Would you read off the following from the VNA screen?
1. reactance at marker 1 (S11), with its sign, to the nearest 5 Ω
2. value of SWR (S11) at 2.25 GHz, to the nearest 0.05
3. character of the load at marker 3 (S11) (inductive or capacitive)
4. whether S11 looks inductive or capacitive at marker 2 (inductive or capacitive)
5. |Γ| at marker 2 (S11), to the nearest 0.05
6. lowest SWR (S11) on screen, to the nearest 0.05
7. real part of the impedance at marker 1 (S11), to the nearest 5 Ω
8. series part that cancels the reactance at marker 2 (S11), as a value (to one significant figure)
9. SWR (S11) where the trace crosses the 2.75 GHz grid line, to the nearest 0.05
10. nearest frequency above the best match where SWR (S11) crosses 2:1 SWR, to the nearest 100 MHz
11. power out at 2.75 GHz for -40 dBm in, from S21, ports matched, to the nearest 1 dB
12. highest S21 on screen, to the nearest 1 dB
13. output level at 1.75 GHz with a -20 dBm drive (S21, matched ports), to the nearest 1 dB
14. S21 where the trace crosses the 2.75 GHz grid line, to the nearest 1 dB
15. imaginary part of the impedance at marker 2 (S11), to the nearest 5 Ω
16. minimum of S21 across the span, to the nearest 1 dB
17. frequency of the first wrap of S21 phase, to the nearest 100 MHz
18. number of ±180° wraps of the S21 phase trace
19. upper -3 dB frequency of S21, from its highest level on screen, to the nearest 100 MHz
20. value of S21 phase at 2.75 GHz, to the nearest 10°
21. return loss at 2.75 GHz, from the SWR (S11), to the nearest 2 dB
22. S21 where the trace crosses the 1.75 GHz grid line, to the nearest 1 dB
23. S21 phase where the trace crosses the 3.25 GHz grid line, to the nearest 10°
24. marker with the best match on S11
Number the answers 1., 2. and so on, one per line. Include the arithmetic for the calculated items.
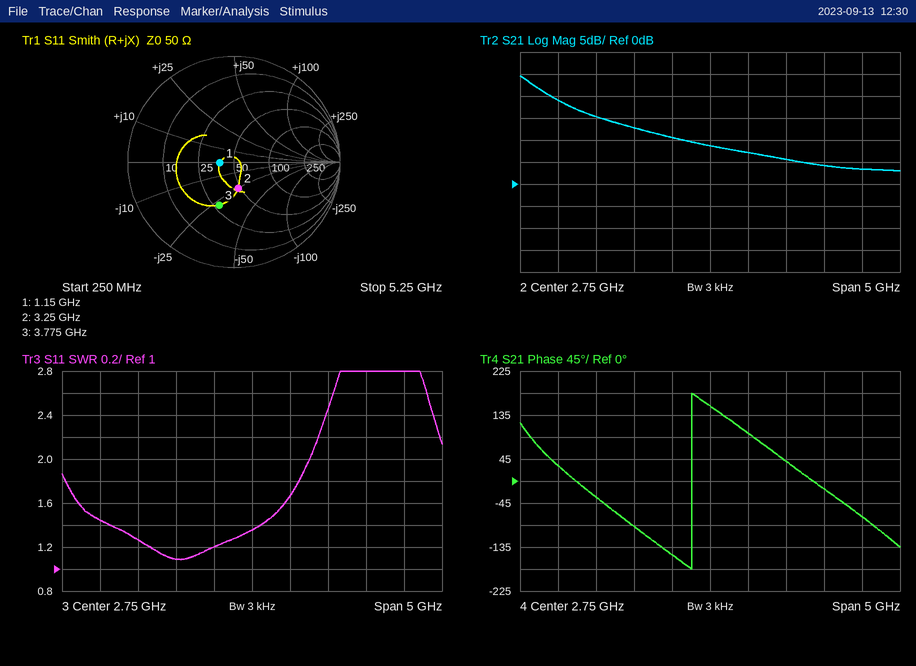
1. 0 Ω
2. 1.20
3. capacitive
4. capacitive
5. 0.25
6. 1.10
7. 40 Ω
8. L = 25 Ω/(2π × 3.25 GHz) ≈ 1 nH
9. 1.35
10. 3.5 GHz
11. -40 dBm + (9 dB) = -31 dBm
12. 25 dB
13. -20 dBm + (13 dB) = -7 dBm
14. 9 dB
15. -25 Ω
16. 3 dB
17. 2.5 GHz
18. 1
19. 500 MHz
20. 150°
21. −20 log10((1.35 − 1)/(1.35 + 1)) ≈ 16 dB
22. 13 dB
23. 100°
24. marker 1
